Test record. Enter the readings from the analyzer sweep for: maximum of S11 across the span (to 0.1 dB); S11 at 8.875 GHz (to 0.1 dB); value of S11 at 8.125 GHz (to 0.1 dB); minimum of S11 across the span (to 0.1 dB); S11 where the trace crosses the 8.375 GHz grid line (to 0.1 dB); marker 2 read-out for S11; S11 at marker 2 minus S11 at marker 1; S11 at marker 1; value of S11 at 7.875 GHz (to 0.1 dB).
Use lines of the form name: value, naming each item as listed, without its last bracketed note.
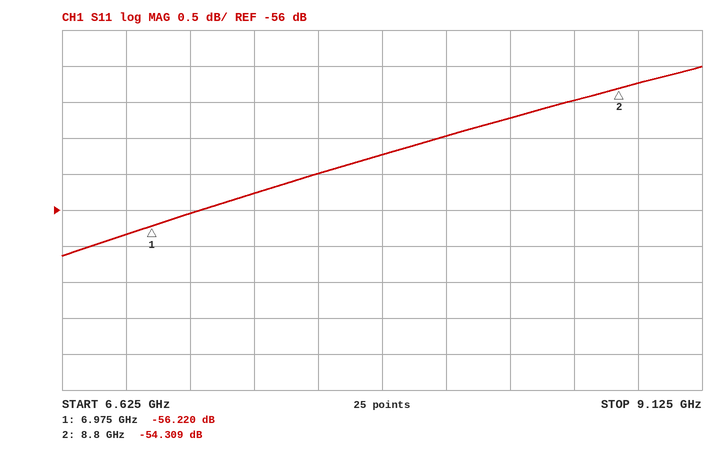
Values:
maximum of S11 across the span: -54.0 dB
S11 at 8.875 GHz: -54.2 dB
value of S11 at 8.125 GHz: -55.0 dB
minimum of S11 across the span: -56.6 dB
S11 where the trace crosses the 8.375 GHz grid line: -54.7 dB
marker 2 read-out for S11: -54.309 dB
S11 at marker 2 minus S11 at marker 1: 1.911 dB
S11 at marker 1: -56.220 dB
value of S11 at 7.875 GHz: -55.2 dB
